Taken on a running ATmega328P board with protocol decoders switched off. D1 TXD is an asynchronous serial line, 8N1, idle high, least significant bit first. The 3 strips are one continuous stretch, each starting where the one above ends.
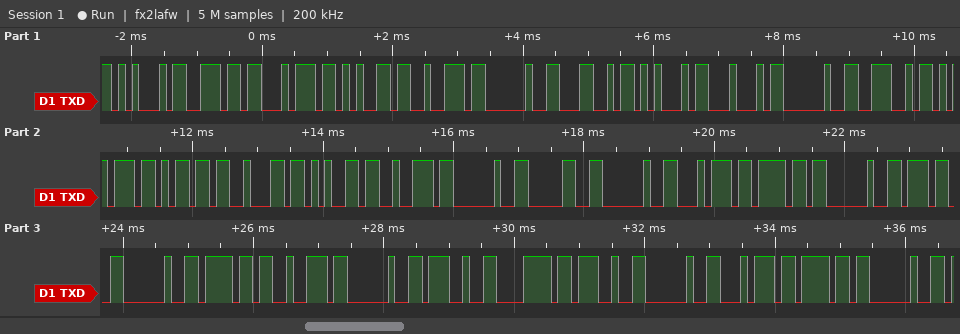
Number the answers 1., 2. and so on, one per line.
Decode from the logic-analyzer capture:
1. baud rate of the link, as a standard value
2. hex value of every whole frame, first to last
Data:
1. 9600 baud
2. 45 6E 74 65 72 20 4C 45 44 20 4E 75 6D 62 65 72 20 30 20 74 6F 20 37 20 6F 72 20 27 78 27 20 74 6F 20
